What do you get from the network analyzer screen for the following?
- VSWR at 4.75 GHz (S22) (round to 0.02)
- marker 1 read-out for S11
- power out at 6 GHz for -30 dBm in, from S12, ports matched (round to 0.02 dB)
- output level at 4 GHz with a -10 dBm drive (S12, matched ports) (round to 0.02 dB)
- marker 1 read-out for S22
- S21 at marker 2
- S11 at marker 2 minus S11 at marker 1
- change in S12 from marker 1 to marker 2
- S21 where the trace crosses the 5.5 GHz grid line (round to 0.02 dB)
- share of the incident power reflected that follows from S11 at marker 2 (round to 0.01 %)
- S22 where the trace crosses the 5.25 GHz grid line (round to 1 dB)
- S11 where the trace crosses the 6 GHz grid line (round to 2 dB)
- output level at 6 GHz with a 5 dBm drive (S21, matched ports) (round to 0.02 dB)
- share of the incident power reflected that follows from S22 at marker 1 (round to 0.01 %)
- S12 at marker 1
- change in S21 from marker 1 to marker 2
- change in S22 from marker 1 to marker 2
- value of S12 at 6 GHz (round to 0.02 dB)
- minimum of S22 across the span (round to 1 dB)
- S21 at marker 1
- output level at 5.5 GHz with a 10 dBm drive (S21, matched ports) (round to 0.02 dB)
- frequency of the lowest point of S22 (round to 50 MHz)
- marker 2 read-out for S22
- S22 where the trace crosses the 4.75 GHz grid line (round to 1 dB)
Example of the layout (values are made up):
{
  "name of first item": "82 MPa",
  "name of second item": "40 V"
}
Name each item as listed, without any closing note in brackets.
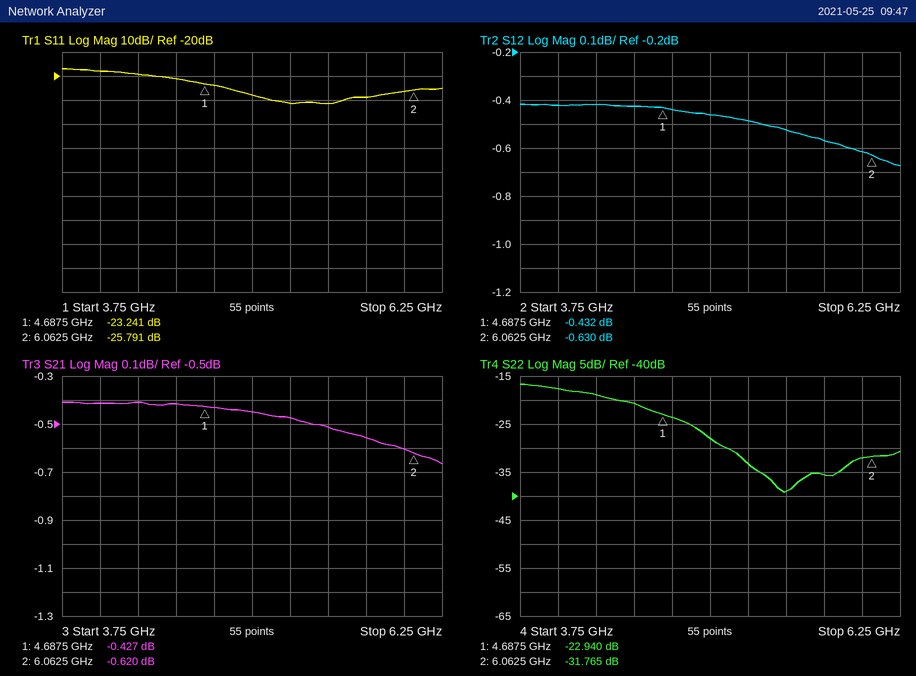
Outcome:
{
  "VSWR at 4.75 GHz (S22)": "1.14",
  "marker 1 read-out for S11": "-23.241 dB",
  "power out at 6 GHz for -30 dBm in, from S12, ports matched": "-30.62 dBm",
  "output level at 4 GHz with a -10 dBm drive (S12, matched ports)": "-10.42 dBm",
  "marker 1 read-out for S22": "-22.940 dB",
  "S21 at marker 2": "-0.620 dB",
  "S11 at marker 2 minus S11 at marker 1": "-2.550 dB",
  "change in S12 from marker 1 to marker 2": "-0.198 dB",
  "S21 where the trace crosses the 5.5 GHz grid line": "-0.52 dB",
  "share of the incident power reflected that follows from S11 at marker 2": "0.26 %",
  "S22 where the trace crosses the 5.25 GHz grid line": "-33 dB",
  "S11 where the trace crosses the 6 GHz grid line": "-26 dB",
  "output level at 6 GHz with a 5 dBm drive (S21, matched ports)": "4.40 dBm",
  "share of the incident power reflected that follows from S22 at marker 1": "0.51 %",
  "S12 at marker 1": "-0.432 dB",
  "change in S21 from marker 1 to marker 2": "-0.193 dB",
  "change in S22 from marker 1 to marker 2": "-8.825 dB",
  "value of S12 at 6 GHz": "-0.62 dB",
  "minimum of S22 across the span": "-39 dB",
  "S21 at marker 1": "-0.427 dB",
  "output level at 5.5 GHz with a 10 dBm drive (S21, matched ports)": "9.48 dBm",
  "frequency of the lowest point of S22": "5.50 GHz",
  "marker 2 read-out for S22": "-31.765 dB",
  "S22 where the trace crosses the 4.75 GHz grid line": "-24 dB"
}
